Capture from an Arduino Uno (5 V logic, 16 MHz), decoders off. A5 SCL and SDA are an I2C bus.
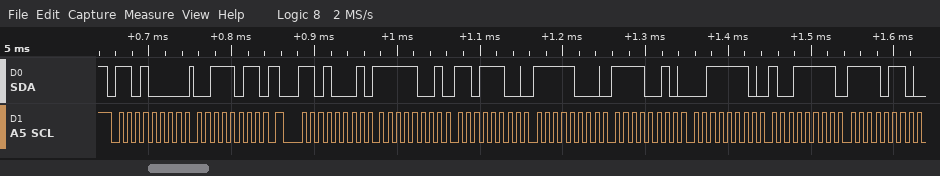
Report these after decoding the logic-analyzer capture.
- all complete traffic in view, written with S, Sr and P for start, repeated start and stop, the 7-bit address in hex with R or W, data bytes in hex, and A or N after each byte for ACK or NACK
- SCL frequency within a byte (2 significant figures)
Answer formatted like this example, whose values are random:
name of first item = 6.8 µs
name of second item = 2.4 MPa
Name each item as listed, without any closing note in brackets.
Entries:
all complete traffic in view, written with S, Sr and P for start, repeated start and stop, the 7-bit address in hex with R or W, data bytes in hex, and A or N after each byte for ACK or NACK = S 68W A 3B A Sr 68R A F9 A DC A F8 A F2 A 3E A 9F A F6 A
SCL frequency within a byte = 100 kHz
